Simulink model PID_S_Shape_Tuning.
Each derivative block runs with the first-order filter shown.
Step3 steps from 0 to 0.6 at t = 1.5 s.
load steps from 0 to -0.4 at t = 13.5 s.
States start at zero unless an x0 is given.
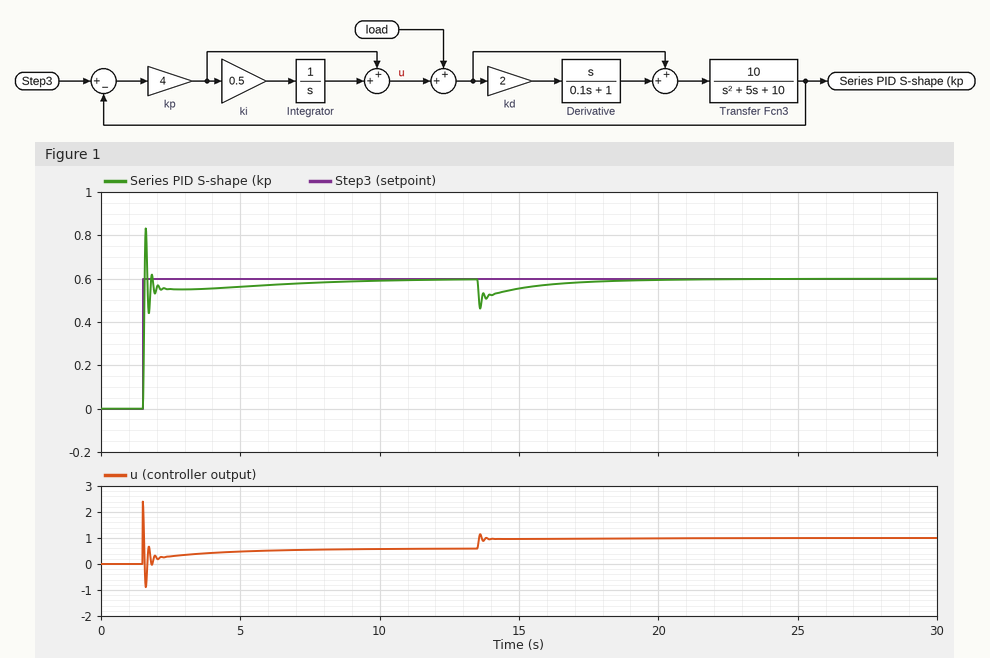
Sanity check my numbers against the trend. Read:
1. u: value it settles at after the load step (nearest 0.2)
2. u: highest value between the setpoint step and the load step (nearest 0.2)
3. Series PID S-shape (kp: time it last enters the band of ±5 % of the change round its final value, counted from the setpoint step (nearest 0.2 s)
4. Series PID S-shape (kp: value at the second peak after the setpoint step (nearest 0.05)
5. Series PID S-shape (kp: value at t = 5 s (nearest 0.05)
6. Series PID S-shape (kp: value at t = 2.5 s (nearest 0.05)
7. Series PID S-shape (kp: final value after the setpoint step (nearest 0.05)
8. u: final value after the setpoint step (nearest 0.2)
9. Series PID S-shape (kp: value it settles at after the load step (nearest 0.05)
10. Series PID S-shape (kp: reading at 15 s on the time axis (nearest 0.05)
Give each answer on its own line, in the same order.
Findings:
1.0
2.4
4.4 s
0.60
0.55
0.55
0.60
0.6
0.60
0.55
